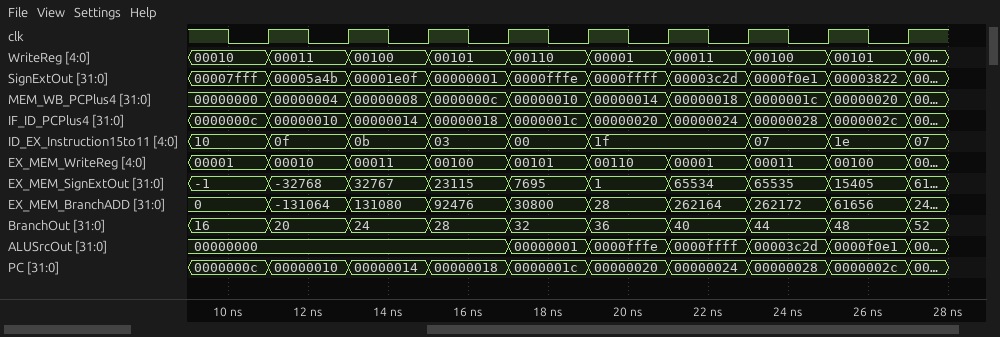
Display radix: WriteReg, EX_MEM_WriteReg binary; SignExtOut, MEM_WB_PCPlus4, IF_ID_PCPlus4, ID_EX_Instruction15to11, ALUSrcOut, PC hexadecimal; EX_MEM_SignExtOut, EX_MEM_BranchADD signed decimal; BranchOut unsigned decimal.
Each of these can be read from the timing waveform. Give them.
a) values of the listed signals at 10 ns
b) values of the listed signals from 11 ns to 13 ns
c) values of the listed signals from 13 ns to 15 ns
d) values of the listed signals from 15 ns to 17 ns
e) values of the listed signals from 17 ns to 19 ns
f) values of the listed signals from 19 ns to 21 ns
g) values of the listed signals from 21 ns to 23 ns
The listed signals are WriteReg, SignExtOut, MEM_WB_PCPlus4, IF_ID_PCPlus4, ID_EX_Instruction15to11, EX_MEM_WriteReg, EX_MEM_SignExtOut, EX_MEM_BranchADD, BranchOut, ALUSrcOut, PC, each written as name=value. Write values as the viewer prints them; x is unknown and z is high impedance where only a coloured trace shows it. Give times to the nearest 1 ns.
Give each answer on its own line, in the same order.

WriteReg=00010, SignExtOut=00007fff, MEM_WB_PCPlus4=00000000, IF_ID_PCPlus4=0000000c, ID_EX_Instruction15to11=10, EX_MEM_WriteReg=00001, EX_MEM_SignExtOut=-1, EX_MEM_BranchADD=0, BranchOut=16, ALUSrcOut=00000000, PC=0000000c
WriteReg=00011, SignExtOut=00005a4b, MEM_WB_PCPlus4=00000004, IF_ID_PCPlus4=00000010, ID_EX_Instruction15to11=0f, EX_MEM_WriteReg=00010, EX_MEM_SignExtOut=-32768, EX_MEM_BranchADD=-131064, BranchOut=20, ALUSrcOut=00000000, PC=00000010
WriteReg=00100, SignExtOut=00001e0f, MEM_WB_PCPlus4=00000008, IF_ID_PCPlus4=00000014, ID_EX_Instruction15to11=0b, EX_MEM_WriteReg=00011, EX_MEM_SignExtOut=32767, EX_MEM_BranchADD=131080, BranchOut=24, ALUSrcOut=00000000, PC=00000014
WriteReg=00101, SignExtOut=00000001, MEM_WB_PCPlus4=0000000c, IF_ID_PCPlus4=00000018, ID_EX_Instruction15to11=03, EX_MEM_WriteReg=00100, EX_MEM_SignExtOut=23115, EX_MEM_BranchADD=92476, BranchOut=28, ALUSrcOut=00000000, PC=00000018
WriteReg=00110, SignExtOut=0000fffe, MEM_WB_PCPlus4=00000010, IF_ID_PCPlus4=0000001c, ID_EX_Instruction15to11=00, EX_MEM_WriteReg=00101, EX_MEM_SignExtOut=7695, EX_MEM_BranchADD=30800, BranchOut=32, ALUSrcOut=00000001, PC=0000001c
WriteReg=00001, SignExtOut=0000ffff, MEM_WB_PCPlus4=00000014, IF_ID_PCPlus4=00000020, ID_EX_Instruction15to11=1f, EX_MEM_WriteReg=00110, EX_MEM_SignExtOut=1, EX_MEM_BranchADD=28, BranchOut=36, ALUSrcOut=0000fffe, PC=00000020
WriteReg=00011, SignExtOut=00003c2d, MEM_WB_PCPlus4=00000018, IF_ID_PCPlus4=00000024, ID_EX_Instruction15to11=1f, EX_MEM_WriteReg=00001, EX_MEM_SignExtOut=65534, EX_MEM_BranchADD=262164, BranchOut=40, ALUSrcOut=0000ffff, PC=00000024
